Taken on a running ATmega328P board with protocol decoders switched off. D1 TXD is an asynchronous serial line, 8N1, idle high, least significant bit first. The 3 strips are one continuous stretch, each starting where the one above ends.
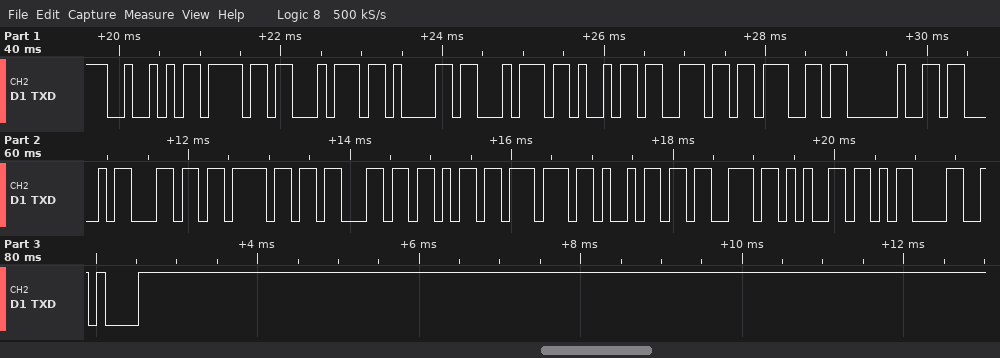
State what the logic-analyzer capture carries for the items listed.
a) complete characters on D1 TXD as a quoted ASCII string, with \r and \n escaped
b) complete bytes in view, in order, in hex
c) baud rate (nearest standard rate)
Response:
"Rotating Clockwise\r\n"
52 6F 74 61 74 69 6E 67 20 43 6C 6F 63 6B 77 69 73 65 0D 0A
9600 baud
